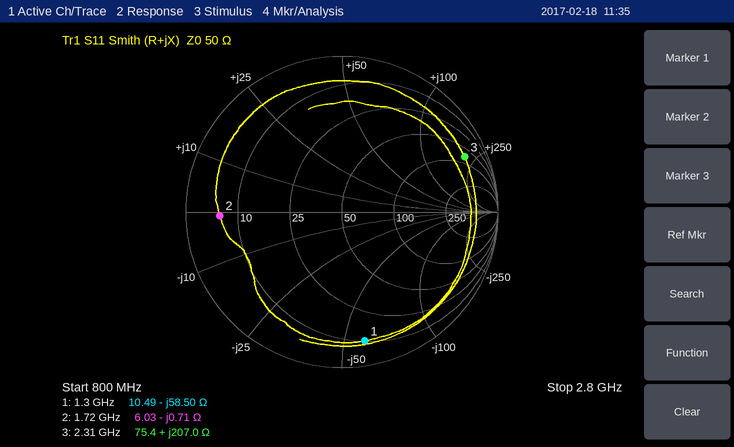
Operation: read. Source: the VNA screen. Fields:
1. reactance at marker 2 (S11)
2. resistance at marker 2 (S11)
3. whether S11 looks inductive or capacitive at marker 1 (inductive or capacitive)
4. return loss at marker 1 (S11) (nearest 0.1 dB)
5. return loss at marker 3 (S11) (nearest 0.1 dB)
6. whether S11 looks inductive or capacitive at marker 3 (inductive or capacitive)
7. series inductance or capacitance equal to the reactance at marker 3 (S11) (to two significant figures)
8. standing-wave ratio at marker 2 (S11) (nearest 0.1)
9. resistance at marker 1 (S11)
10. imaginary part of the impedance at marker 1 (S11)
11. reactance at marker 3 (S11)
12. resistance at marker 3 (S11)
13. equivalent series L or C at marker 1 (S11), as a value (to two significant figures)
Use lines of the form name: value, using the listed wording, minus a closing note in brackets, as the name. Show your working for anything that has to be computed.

reactance at marker 2: -0.71 Ω
resistance at marker 2: 6.03 Ω
whether S11 looks inductive or capacitive at marker 1: capacitive
return loss at marker 1 (S11): 1.5 dB
return loss at marker 3 (S11): 1.3 dB
whether S11 looks inductive or capacitive at marker 3: inductive
series inductance or capacitance equal to the reactance at marker 3 (S11): L = 207 Ω/(2π × 2.31 GHz) ≈ 14 nH
standing-wave ratio at marker 2 (S11): 8.3
resistance at marker 1: 10.49 Ω
imaginary part of the impedance at marker 1: -58.50 Ω
reactance at marker 3: +207.0 Ω
resistance at marker 3: 75.4 Ω
equivalent series L or C at marker 1 (S11), as a value: C = 1/(2π × 1.3 GHz × 58.5 Ω) ≈ 2.1 pF
